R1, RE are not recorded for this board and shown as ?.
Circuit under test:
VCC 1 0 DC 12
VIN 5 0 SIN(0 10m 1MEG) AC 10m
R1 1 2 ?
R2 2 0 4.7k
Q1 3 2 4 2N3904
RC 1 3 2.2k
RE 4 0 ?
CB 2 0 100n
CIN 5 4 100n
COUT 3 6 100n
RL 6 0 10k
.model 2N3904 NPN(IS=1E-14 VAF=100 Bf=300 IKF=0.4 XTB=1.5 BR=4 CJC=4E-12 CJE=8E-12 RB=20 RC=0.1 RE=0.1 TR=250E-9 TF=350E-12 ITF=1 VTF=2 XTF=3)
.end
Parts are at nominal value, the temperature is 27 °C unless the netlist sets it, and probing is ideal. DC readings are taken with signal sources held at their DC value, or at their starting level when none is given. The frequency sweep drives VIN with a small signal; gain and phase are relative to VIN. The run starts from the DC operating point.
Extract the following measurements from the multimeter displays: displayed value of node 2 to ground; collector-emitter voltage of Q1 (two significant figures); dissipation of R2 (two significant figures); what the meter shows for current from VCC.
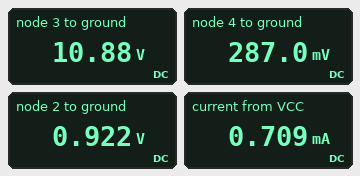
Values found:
0.922 V
11 V
180 µW
0.709 mA
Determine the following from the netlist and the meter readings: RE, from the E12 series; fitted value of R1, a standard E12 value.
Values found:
560 Ω
56 kΩ
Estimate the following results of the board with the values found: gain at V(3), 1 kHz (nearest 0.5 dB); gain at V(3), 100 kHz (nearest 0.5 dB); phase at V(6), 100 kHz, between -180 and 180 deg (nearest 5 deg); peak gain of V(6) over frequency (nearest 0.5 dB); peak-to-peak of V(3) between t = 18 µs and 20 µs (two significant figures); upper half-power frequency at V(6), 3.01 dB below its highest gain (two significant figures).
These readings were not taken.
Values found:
0.5 dB
30.5 dB
20 deg
31.0 dB
700 mV
37 MHz
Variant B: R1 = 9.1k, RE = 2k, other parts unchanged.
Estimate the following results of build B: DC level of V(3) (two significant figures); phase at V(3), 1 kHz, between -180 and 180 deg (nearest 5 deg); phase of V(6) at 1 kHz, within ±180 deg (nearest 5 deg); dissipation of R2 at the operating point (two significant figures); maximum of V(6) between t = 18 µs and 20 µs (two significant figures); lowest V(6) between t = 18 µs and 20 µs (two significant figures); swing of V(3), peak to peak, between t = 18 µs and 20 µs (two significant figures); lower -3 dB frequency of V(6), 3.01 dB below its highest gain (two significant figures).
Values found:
8.3 V
90 deg
95 deg
3.5 mW
1.0 V
-1.2 V
2.2 V
100 kHz
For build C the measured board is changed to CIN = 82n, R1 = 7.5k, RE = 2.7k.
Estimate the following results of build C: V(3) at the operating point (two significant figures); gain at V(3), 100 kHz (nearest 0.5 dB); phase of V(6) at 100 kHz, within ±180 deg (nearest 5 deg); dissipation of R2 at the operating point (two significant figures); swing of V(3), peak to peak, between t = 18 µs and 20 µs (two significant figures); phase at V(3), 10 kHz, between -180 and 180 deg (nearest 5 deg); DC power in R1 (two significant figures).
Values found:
8.8 V
36.5 dB
45 deg
4.5 mW
1.9 V
85 deg
7.3 mW
